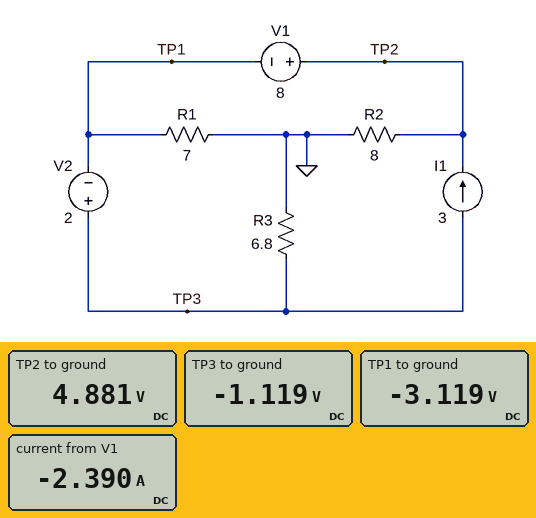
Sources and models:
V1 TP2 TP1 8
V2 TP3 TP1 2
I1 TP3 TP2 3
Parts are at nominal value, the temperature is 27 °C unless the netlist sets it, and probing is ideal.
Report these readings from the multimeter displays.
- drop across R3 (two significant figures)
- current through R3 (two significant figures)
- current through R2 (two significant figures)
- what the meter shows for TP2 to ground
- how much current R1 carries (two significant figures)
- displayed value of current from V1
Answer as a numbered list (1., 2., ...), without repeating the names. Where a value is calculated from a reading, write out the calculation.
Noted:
1. 0 V - (-1.119 V) = 1.1 V
2. (0 V - (-1.119 V)) / 6.8 Ω = 160 mA
3. (4.881 V) / 8 Ω = 610 mA
4. 4.881 V
5. (0 V - (-3.119 V)) / 7 Ω = 450 mA
6. -2.390 A
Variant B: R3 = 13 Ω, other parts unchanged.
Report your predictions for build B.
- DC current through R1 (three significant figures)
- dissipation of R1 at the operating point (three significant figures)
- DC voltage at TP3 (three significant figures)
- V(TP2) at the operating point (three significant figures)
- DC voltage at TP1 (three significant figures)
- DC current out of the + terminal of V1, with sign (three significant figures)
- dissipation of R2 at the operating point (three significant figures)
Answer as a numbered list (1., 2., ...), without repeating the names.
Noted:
1. 478 mA
2. 1.60 W
3. -1.35 V
4. 4.65 V
5. -3.35 V
6. -2.42 A
7. 2.71 W
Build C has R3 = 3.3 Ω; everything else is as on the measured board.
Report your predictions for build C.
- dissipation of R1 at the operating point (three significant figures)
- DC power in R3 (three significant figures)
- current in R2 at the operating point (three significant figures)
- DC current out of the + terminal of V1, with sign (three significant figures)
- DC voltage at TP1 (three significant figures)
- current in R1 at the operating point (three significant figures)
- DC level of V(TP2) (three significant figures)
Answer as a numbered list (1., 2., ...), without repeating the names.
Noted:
1. 1.13 W
2. 200 mW
3. 648 mA
4. -2.35 A
5. -2.81 V
6. 402 mA
7. 5.19 V
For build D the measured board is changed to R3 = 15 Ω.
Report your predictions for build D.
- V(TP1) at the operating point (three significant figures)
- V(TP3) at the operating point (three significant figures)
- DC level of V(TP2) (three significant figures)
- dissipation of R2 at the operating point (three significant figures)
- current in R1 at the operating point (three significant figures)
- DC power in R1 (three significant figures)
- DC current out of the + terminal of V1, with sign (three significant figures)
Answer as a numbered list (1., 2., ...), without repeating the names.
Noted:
1. -3.39 V
2. -1.39 V
3. 4.61 V
4. 2.66 W
5. 484 mA
6. 1.64 W
7. -2.42 A
